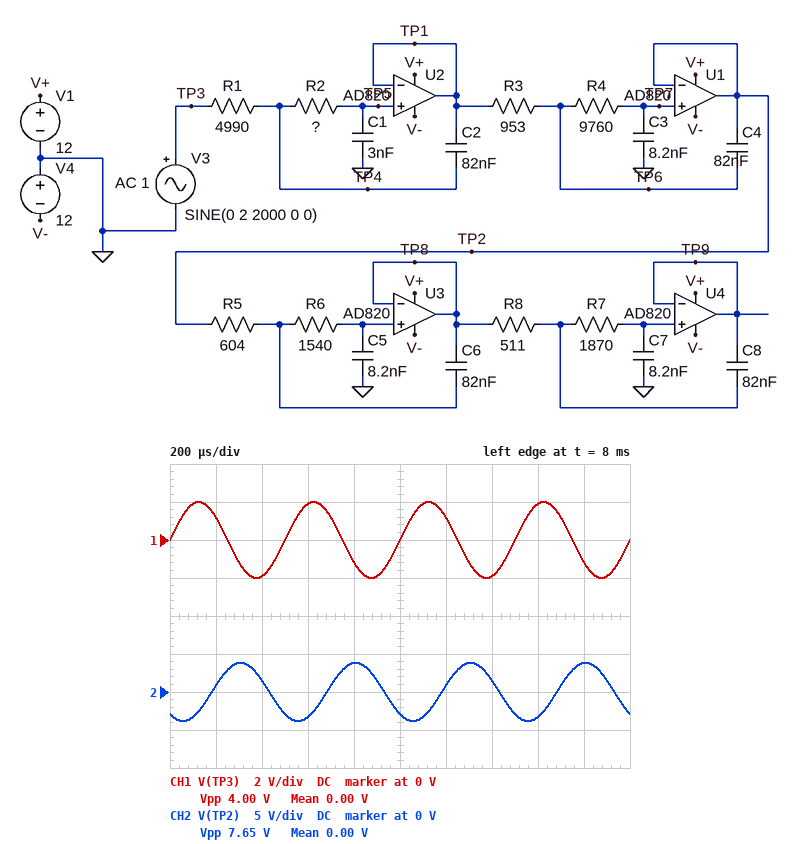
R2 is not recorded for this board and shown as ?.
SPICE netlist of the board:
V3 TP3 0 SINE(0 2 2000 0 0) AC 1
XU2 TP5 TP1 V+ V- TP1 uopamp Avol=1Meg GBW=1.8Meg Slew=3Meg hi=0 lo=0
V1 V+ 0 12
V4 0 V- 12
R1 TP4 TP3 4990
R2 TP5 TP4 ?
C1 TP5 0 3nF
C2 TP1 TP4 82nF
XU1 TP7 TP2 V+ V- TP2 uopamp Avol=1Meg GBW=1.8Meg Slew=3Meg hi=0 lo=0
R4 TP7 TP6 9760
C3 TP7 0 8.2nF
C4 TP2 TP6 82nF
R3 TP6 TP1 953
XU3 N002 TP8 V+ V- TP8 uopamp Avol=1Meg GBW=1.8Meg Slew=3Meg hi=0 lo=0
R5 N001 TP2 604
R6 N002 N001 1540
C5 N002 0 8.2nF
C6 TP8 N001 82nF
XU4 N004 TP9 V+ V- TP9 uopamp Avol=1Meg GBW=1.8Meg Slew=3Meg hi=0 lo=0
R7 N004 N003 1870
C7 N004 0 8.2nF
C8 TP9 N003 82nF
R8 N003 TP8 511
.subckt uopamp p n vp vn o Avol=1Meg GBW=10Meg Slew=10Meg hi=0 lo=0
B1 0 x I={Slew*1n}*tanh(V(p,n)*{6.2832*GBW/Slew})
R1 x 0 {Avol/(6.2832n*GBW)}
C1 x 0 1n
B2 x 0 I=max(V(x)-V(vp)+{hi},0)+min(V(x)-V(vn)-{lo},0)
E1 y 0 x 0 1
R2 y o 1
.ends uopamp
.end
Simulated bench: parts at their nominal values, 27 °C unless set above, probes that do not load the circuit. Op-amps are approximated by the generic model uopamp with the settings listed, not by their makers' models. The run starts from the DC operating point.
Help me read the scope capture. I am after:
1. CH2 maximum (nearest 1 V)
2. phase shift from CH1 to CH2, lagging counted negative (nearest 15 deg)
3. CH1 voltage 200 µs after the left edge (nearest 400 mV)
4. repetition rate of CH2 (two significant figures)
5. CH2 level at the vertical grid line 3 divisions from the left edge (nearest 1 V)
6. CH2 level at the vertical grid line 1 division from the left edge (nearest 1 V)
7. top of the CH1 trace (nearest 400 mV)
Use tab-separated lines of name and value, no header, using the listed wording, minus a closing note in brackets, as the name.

CH2 maximum	4 V
phase shift from CH1 to CH2, lagging counted negative	-135 deg
CH1 voltage 200 µs after the left edge	1.2 V
repetition rate of CH2	2.0 kHz
CH2 level at the vertical grid line 3 divisions from the left edge	-3 V
CH2 level at the vertical grid line 1 division from the left edge	1 V
top of the CH1 trace	2.0 V
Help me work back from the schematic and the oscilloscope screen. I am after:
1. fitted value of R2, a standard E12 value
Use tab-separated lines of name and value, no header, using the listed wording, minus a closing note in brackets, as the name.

fitted value of R2, a standard E12 value	3.3 kΩ
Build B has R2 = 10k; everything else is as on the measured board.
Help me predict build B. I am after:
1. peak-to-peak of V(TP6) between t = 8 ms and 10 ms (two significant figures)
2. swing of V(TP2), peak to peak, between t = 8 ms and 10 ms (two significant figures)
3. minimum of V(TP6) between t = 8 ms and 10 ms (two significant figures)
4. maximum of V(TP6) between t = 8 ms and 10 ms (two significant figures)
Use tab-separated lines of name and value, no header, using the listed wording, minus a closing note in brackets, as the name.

peak-to-peak of V(TP6) between t = 8 ms and 10 ms	4.7 V
swing of V(TP2), peak to peak, between t = 8 ms and 10 ms	3.3 V
minimum of V(TP6) between t = 8 ms and 10 ms	-2.3 V
maximum of V(TP6) between t = 8 ms and 10 ms	2.3 V
